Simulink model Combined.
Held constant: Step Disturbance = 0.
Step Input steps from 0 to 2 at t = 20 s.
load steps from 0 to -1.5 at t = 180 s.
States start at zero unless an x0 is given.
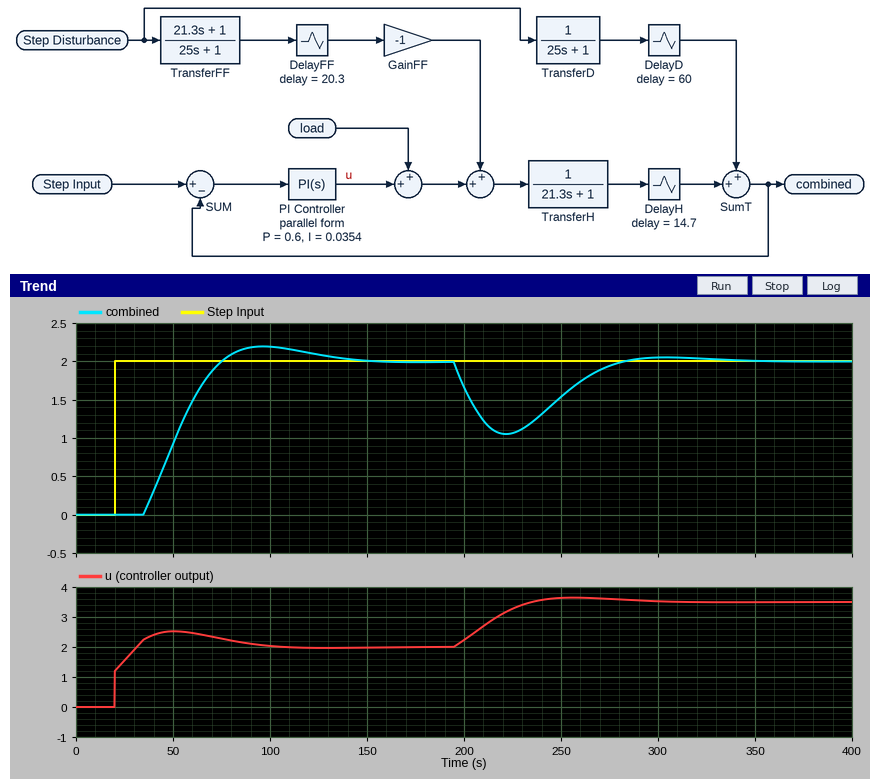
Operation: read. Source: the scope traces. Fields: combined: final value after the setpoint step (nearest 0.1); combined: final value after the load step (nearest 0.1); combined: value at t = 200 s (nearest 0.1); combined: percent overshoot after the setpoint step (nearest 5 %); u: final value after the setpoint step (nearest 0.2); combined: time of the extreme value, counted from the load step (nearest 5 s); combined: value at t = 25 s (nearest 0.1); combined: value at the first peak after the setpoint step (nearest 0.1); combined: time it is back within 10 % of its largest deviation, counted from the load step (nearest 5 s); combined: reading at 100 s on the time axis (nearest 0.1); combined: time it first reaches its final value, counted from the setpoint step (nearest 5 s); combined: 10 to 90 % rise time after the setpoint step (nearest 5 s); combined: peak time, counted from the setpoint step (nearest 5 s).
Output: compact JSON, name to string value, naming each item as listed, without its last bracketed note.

{"combined: final value after the setpoint step": "2.0", "combined: final value after the load step": "2.0", "combined: value at t = 200 s": "1.7", "combined: percent overshoot after the setpoint step": "10 %", "u: final value after the setpoint step": "2.0", "combined: time of the extreme value, counted from the load step": "40 s", "combined: value at t = 25 s": "0.0", "combined: value at the first peak after the setpoint step": "2.2", "combined: time it is back within 10 % of its largest deviation, counted from the load step": "90 s", "combined: reading at 100 s on the time axis": "2.2", "combined: time it first reaches its final value, counted from the setpoint step": "55 s", "combined: 10 to 90 % rise time after the setpoint step": "30 s", "combined: peak time, counted from the setpoint step": "75 s"}
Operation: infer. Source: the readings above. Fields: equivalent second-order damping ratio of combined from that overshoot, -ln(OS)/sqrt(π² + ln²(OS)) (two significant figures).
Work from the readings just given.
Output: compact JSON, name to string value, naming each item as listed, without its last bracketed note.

{"equivalent second-order damping ratio of combined from that overshoot, -ln(OS)/sqrt(π² + ln²(OS))": "0.59"}
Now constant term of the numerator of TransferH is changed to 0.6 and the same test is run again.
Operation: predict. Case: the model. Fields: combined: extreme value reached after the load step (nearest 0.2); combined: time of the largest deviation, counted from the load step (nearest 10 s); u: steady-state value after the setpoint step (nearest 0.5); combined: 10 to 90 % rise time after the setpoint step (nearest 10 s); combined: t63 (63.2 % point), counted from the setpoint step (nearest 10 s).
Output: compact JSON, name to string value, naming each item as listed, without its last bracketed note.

{"combined: extreme value reached after the load step": "1.4", "combined: time of the largest deviation, counted from the load step": "50 s", "u: steady-state value after the setpoint step": "3.5", "combined: 10 to 90 % rise time after the setpoint step": "60 s", "combined: t63 (63.2 % point), counted from the setpoint step": "50 s"}
